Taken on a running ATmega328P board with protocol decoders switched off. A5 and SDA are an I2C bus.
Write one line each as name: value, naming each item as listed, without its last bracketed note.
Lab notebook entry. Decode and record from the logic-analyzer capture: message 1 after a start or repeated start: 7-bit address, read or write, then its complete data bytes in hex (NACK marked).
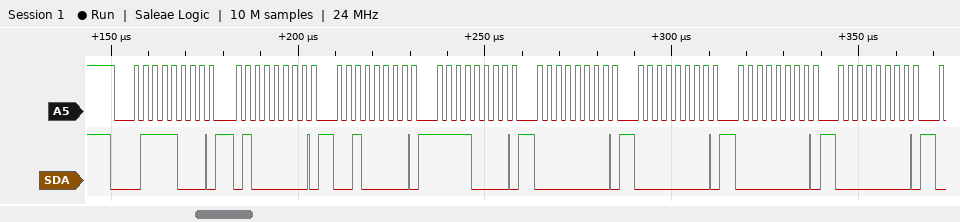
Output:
message 1 after a start or repeated start: 7-bit address, read or write, then its complete data bytes in hex: 0x3C write: 40 20 F0 00 00 00 00
